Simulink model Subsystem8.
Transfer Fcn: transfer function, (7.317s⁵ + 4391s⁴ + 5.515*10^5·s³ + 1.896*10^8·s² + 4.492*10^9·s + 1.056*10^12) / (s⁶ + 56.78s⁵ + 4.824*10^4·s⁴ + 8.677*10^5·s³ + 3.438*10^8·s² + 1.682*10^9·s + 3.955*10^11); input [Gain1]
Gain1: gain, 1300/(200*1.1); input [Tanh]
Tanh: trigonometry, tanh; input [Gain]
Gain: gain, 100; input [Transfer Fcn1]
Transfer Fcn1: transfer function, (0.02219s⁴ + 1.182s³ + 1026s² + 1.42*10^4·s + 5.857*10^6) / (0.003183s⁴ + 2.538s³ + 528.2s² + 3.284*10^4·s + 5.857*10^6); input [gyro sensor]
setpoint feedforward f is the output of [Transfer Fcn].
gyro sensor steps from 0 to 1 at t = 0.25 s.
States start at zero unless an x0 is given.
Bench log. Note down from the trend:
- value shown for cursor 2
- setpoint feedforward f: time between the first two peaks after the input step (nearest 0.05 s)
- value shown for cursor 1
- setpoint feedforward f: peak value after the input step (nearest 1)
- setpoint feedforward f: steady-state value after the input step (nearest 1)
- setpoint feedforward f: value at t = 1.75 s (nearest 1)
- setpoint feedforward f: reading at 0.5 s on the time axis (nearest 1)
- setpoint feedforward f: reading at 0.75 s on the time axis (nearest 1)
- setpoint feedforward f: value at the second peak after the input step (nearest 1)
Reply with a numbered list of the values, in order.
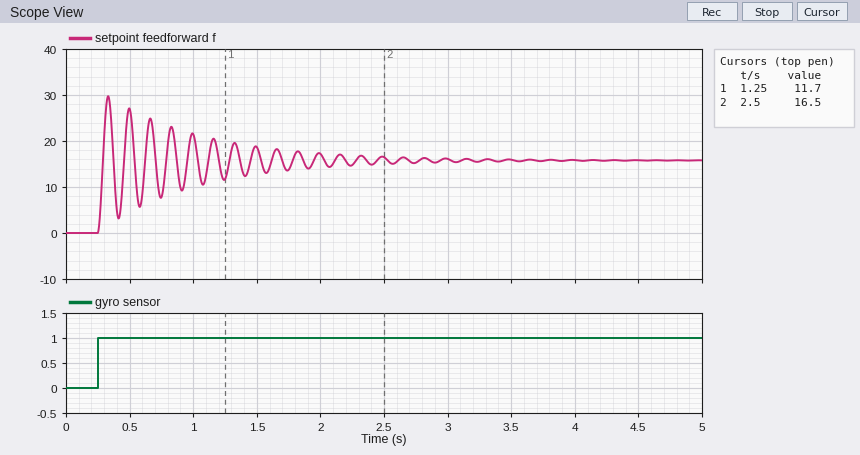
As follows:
1. 16.5
2. 0.15 s
3. 11.7
4. 30
5. 16
6. 14
7. 27
8. 8
9. 27
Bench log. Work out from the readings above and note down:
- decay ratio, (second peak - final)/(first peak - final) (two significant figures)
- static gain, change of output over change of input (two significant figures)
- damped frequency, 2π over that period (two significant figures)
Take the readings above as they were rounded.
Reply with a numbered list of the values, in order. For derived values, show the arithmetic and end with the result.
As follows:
1. (27 - 16) / (30 - 16) = 0.79
2. (16 - 0) / (1 - 0) = 16
3. 2π / 0.15 = 42 rad/s
